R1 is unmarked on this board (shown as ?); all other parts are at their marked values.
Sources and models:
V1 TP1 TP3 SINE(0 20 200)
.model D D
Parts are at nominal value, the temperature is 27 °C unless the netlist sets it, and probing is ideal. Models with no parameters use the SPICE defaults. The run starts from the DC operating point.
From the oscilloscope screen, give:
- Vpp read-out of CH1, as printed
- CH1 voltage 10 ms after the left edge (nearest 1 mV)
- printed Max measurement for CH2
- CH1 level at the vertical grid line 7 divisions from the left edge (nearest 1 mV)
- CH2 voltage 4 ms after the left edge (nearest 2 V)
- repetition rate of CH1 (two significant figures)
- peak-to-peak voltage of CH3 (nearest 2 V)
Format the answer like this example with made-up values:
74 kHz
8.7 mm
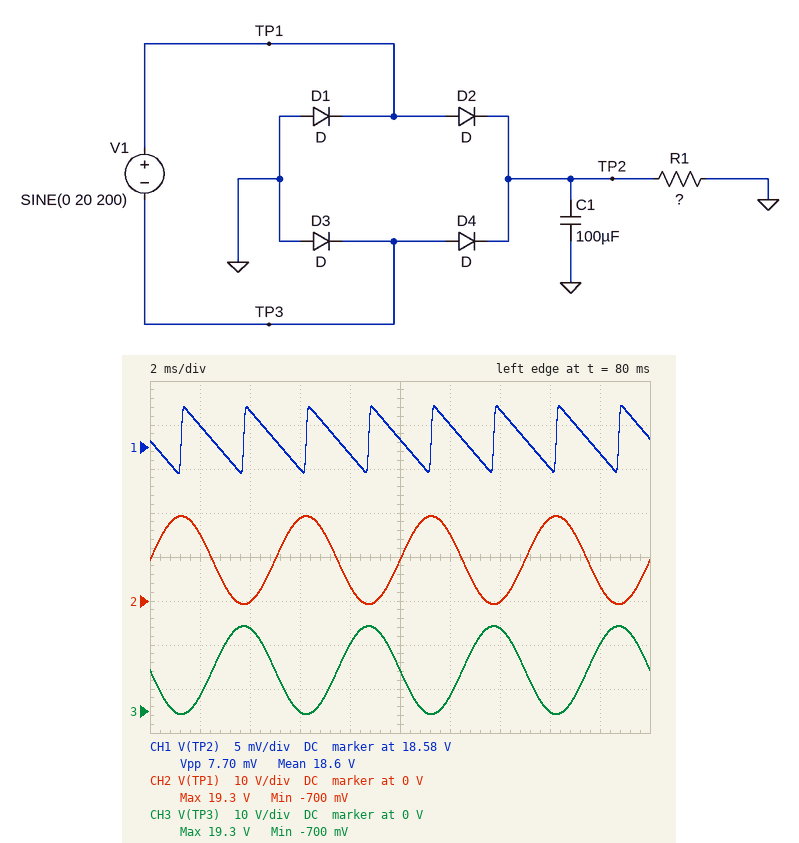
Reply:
7.70 mV
18.581 V
19.3 V
18.584 V
0 V
400 Hz
20 V
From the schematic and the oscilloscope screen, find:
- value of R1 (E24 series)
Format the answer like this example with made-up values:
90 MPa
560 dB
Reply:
56 kΩ
